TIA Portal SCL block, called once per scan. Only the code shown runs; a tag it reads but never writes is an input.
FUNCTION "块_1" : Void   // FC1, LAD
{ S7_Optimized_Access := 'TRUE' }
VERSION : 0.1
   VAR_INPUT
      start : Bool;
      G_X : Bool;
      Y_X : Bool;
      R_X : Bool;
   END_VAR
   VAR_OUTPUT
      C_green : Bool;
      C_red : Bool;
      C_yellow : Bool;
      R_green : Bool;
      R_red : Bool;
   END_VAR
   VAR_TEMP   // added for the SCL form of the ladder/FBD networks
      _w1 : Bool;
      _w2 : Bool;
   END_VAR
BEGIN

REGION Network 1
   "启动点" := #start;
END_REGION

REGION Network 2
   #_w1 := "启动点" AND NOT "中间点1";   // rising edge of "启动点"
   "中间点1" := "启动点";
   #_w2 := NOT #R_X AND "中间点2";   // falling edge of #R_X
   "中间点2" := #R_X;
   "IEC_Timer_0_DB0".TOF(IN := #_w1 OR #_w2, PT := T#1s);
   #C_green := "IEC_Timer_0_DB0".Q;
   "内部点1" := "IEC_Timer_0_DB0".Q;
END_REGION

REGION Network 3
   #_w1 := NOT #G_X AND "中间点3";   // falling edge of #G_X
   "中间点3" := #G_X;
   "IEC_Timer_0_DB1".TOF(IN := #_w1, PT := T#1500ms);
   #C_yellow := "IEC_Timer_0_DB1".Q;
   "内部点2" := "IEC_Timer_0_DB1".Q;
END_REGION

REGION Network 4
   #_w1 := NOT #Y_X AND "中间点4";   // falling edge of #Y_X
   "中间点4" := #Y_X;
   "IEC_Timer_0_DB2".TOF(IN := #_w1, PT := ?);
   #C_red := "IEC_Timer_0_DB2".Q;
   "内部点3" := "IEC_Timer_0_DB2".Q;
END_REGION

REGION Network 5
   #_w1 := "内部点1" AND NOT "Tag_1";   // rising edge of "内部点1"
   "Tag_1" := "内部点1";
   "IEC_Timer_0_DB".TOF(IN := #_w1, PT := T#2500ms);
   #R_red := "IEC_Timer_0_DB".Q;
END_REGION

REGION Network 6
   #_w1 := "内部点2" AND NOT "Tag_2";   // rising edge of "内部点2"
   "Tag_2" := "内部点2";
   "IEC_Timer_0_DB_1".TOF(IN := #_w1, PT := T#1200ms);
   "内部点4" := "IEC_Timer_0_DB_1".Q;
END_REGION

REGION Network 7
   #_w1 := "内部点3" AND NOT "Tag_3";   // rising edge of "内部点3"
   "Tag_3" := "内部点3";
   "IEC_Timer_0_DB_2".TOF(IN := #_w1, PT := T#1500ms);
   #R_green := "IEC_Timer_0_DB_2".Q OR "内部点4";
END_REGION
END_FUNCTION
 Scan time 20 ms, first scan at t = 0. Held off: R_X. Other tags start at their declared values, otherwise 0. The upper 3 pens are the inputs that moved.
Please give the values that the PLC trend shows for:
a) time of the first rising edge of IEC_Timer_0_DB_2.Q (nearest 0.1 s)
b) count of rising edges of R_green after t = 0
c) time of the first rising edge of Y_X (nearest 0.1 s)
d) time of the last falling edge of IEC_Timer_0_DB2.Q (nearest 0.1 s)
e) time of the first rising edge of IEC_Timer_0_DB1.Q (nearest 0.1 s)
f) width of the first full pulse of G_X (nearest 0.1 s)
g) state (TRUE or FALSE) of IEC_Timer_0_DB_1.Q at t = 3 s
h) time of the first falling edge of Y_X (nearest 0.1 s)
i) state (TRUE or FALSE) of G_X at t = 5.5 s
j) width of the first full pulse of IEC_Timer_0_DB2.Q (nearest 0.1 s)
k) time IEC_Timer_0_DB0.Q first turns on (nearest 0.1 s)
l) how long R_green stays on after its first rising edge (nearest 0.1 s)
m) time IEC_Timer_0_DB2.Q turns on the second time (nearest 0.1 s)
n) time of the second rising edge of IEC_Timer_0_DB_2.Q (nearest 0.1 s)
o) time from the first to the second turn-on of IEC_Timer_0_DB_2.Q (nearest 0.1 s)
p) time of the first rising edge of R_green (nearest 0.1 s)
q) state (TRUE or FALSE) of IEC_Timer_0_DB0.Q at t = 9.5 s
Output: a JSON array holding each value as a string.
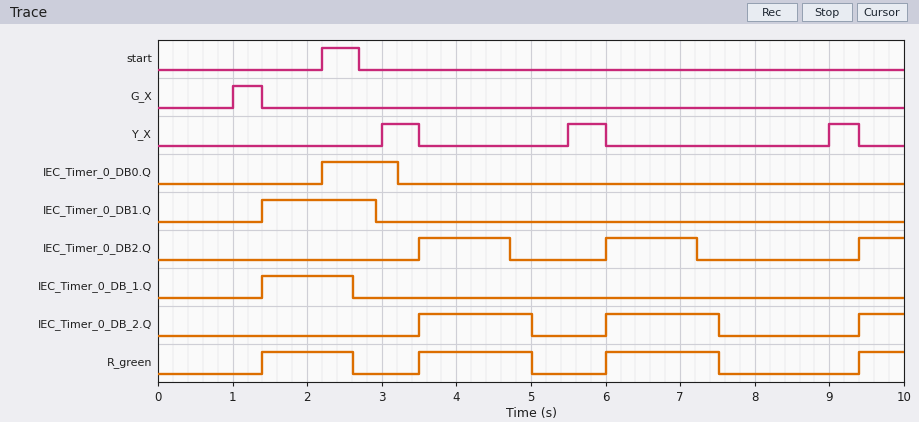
["3.5 s", "4", "3.0 s", "7.2 s", "1.4 s", "0.4 s", "FALSE", "3.5 s", "FALSE", "1.2 s", "2.2 s", "1.2 s", "6.0 s", "6.0 s", "2.5 s", "1.4 s", "FALSE"]
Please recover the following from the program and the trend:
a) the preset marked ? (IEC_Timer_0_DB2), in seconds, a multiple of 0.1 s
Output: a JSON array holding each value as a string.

["1.2 s"]
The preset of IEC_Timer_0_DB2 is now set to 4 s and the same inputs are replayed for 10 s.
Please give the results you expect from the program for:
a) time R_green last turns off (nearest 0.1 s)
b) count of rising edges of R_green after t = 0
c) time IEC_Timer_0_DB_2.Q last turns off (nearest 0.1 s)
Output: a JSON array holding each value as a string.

["5.0 s", "2", "5.0 s"]
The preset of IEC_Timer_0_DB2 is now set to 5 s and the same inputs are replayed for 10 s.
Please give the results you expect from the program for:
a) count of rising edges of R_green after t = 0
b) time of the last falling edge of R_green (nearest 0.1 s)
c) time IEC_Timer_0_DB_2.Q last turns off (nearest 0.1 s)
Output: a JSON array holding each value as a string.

["2", "5.0 s", "5.0 s"]
